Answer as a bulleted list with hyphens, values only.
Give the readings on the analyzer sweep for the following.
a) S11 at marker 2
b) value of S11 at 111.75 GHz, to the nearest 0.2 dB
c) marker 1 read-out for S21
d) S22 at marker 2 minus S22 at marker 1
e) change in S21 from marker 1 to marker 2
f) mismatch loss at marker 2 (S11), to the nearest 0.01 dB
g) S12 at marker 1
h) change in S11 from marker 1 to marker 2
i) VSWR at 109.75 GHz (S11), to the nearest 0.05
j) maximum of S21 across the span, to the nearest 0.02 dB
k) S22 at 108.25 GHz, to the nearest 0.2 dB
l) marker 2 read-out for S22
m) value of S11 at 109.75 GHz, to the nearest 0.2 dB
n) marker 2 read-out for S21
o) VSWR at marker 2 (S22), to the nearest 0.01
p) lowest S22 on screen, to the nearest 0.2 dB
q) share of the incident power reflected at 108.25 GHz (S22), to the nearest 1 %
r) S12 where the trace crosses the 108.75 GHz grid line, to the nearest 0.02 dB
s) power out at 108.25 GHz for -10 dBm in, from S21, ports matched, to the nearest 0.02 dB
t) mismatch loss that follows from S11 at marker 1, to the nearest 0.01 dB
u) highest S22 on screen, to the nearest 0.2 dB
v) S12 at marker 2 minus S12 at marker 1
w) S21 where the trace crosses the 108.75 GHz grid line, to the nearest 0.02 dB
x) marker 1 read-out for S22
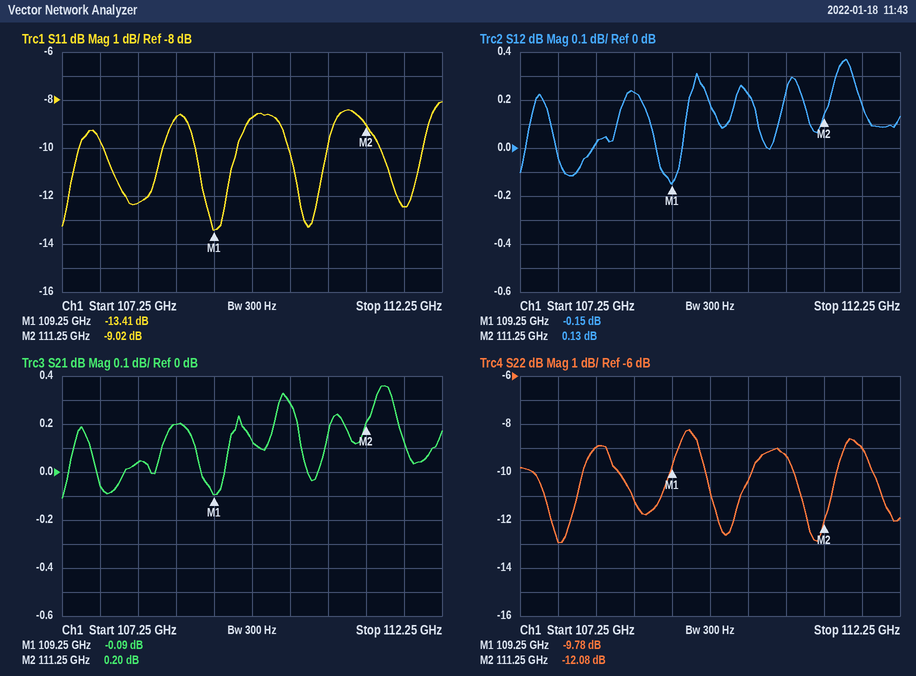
- -9.02 dB
- -12.4 dB
- -0.09 dB
- -2.30 dB
- 0.29 dB
- 0.58 dB
- -0.15 dB
- 4.39 dB
- 2.15
- 0.36 dB
- -9.0 dB
- -12.08 dB
- -8.8 dB
- 0.20 dB
- 1.66
- -13.0 dB
- 13 %
- 0.24 dB
- -9.96 dBm
- 0.20 dB
- -8.2 dB
- 0.28 dB
- 0.20 dB
- -9.78 dB
